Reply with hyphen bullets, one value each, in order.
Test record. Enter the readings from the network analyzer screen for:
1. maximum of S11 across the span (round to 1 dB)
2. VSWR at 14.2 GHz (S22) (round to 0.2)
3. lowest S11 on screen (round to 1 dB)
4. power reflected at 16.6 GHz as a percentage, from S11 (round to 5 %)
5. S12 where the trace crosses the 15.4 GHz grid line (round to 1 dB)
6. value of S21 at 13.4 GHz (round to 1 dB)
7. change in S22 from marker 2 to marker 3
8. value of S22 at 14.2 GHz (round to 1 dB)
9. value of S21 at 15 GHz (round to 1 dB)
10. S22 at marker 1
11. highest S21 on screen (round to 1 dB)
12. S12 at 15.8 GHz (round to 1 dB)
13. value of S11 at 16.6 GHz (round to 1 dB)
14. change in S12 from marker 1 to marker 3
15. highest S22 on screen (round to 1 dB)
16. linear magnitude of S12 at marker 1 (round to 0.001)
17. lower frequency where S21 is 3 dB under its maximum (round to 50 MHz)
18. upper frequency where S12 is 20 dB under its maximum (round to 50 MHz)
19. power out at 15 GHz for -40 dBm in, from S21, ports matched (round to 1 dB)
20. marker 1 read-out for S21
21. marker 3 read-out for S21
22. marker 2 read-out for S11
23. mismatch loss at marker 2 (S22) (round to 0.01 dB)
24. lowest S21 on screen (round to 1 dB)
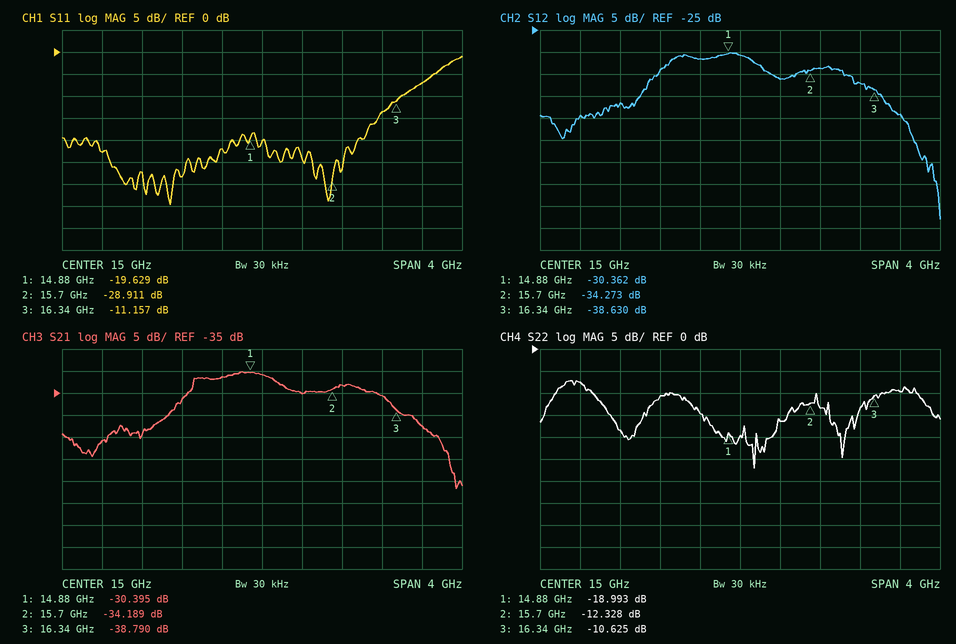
- -1 dB
- 1.8
- -35 dB
- 20 %
- -36 dB
- -46 dB
- 1.703 dB
- -11 dB
- -31 dB
- -18.993 dB
- -30 dB
- -34 dB
- -7 dB
- -8.268 dB
- -7 dB
- 0.030
- 14.30 GHz
- 16.75 GHz
- -71 dBm
- -30.395 dB
- -38.790 dB
- -28.911 dB
- 0.26 dB
- -57 dB
